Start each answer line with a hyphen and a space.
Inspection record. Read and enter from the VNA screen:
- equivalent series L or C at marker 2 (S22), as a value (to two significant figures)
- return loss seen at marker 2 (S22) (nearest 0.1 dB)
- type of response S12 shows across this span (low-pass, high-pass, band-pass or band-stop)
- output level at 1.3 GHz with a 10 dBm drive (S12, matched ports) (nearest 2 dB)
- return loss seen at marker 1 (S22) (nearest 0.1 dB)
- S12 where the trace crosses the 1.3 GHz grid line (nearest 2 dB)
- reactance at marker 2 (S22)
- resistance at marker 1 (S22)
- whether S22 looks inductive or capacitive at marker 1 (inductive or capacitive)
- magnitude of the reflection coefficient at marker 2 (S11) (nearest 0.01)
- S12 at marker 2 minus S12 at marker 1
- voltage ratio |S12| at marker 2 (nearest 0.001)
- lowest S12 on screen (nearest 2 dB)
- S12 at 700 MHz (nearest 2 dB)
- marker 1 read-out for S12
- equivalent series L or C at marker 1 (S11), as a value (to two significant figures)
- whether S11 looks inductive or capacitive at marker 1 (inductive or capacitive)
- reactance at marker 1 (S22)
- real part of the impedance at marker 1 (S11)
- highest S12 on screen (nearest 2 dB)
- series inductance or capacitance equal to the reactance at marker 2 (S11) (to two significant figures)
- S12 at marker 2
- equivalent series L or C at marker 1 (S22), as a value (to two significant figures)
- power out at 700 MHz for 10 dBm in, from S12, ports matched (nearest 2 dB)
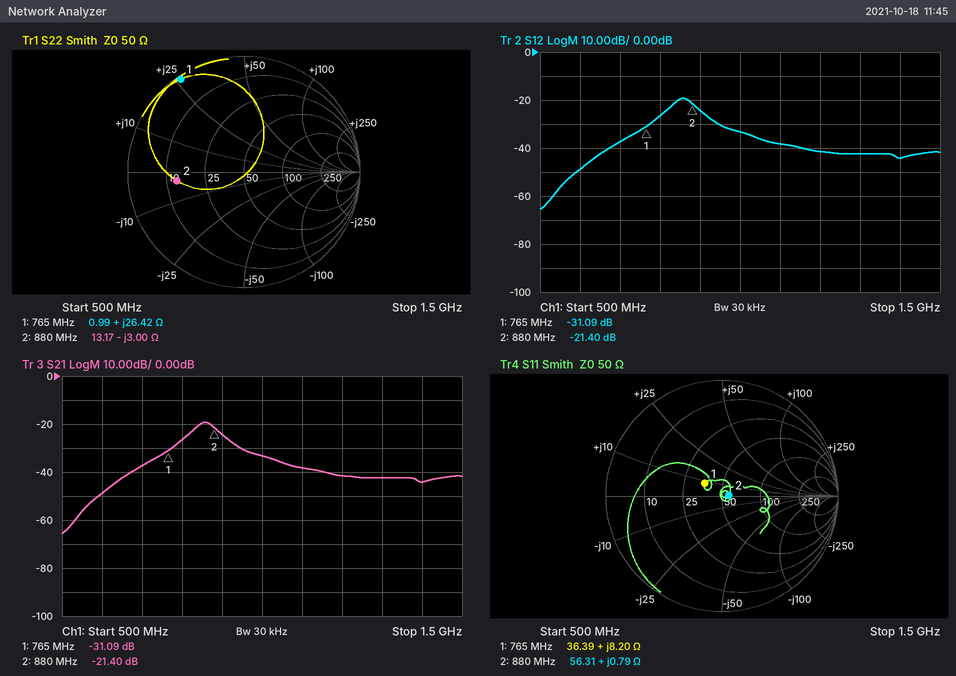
- 60 pF
- 4.7 dB
- band-pass
- -32 dBm
- 0.3 dB
- -42 dB
- -3.00 Ω
- 0.99 Ω
- inductive
- 0.06
- 9.69 dB
- 0.085
- -66 dB
- -38 dB
- -31.09 dB
- 1.7 nH
- inductive
- +26.42 Ω
- 36.39 Ω
- -20 dB
- 140 pH
- -21.40 dB
- 5.5 nH
- -28 dBm
